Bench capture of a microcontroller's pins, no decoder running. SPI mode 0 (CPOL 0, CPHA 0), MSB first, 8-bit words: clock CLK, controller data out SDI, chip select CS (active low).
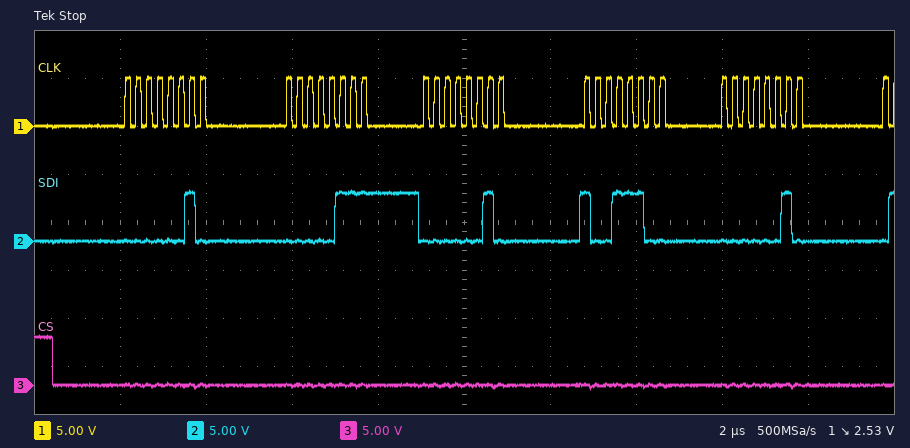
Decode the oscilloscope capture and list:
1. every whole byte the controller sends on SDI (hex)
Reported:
0x02 0x07 0x02 0x9C 0x02
